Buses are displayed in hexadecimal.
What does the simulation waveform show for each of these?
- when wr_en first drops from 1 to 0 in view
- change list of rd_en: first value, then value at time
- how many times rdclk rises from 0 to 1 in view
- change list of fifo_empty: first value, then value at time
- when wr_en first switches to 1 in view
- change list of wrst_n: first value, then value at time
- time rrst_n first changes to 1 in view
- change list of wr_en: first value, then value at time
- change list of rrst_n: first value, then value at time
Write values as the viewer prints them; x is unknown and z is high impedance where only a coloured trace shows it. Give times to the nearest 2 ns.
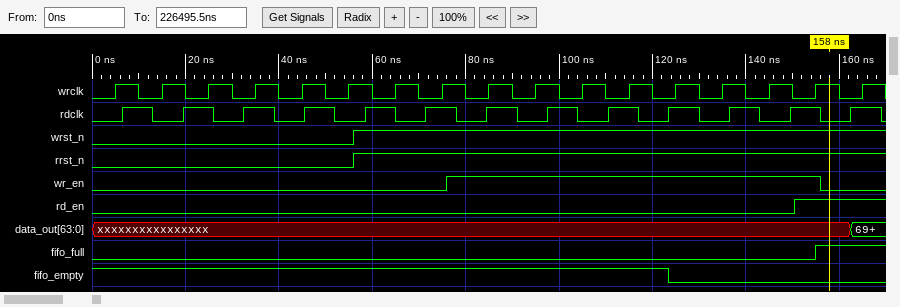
156 ns
0, 1 at 150 ns
13
1, 0 at 124 ns
76 ns
0, 1 at 56 ns
56 ns
0, 1 at 76 ns, 0 at 156 ns
0, 1 at 56 ns
